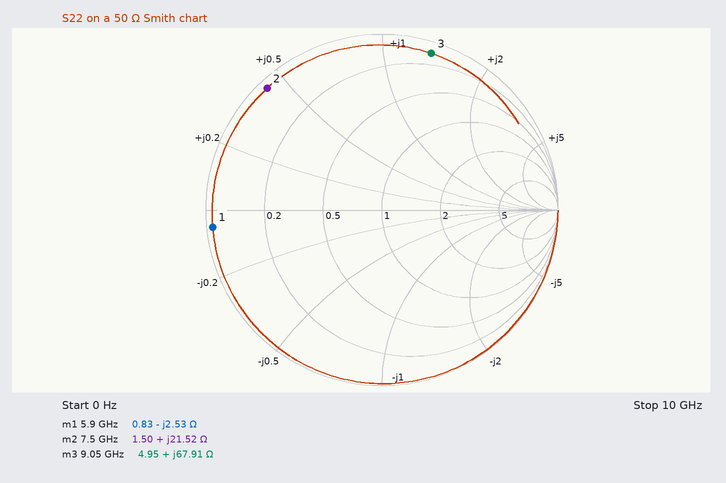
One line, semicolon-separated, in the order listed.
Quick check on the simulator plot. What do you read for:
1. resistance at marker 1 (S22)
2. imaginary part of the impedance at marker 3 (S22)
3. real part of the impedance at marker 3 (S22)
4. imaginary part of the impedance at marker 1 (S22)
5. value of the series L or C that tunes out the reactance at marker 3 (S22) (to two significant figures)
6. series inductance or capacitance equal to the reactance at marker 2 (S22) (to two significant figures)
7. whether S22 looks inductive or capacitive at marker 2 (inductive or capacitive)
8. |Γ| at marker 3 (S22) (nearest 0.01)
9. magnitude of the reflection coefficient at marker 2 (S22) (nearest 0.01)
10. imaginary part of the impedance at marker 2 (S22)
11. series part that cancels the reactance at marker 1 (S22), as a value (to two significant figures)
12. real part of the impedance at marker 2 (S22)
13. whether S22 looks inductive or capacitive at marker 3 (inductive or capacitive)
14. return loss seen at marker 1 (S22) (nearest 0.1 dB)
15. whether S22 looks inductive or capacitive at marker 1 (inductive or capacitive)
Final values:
0.83 Ω; +67.91 Ω; 4.95 Ω; -2.53 Ω; 260 fF; 460 pH; inductive; 0.93; 0.95; +21.52 Ω; 68 pH; 1.50 Ω; inductive; 0.3 dB; capacitive
